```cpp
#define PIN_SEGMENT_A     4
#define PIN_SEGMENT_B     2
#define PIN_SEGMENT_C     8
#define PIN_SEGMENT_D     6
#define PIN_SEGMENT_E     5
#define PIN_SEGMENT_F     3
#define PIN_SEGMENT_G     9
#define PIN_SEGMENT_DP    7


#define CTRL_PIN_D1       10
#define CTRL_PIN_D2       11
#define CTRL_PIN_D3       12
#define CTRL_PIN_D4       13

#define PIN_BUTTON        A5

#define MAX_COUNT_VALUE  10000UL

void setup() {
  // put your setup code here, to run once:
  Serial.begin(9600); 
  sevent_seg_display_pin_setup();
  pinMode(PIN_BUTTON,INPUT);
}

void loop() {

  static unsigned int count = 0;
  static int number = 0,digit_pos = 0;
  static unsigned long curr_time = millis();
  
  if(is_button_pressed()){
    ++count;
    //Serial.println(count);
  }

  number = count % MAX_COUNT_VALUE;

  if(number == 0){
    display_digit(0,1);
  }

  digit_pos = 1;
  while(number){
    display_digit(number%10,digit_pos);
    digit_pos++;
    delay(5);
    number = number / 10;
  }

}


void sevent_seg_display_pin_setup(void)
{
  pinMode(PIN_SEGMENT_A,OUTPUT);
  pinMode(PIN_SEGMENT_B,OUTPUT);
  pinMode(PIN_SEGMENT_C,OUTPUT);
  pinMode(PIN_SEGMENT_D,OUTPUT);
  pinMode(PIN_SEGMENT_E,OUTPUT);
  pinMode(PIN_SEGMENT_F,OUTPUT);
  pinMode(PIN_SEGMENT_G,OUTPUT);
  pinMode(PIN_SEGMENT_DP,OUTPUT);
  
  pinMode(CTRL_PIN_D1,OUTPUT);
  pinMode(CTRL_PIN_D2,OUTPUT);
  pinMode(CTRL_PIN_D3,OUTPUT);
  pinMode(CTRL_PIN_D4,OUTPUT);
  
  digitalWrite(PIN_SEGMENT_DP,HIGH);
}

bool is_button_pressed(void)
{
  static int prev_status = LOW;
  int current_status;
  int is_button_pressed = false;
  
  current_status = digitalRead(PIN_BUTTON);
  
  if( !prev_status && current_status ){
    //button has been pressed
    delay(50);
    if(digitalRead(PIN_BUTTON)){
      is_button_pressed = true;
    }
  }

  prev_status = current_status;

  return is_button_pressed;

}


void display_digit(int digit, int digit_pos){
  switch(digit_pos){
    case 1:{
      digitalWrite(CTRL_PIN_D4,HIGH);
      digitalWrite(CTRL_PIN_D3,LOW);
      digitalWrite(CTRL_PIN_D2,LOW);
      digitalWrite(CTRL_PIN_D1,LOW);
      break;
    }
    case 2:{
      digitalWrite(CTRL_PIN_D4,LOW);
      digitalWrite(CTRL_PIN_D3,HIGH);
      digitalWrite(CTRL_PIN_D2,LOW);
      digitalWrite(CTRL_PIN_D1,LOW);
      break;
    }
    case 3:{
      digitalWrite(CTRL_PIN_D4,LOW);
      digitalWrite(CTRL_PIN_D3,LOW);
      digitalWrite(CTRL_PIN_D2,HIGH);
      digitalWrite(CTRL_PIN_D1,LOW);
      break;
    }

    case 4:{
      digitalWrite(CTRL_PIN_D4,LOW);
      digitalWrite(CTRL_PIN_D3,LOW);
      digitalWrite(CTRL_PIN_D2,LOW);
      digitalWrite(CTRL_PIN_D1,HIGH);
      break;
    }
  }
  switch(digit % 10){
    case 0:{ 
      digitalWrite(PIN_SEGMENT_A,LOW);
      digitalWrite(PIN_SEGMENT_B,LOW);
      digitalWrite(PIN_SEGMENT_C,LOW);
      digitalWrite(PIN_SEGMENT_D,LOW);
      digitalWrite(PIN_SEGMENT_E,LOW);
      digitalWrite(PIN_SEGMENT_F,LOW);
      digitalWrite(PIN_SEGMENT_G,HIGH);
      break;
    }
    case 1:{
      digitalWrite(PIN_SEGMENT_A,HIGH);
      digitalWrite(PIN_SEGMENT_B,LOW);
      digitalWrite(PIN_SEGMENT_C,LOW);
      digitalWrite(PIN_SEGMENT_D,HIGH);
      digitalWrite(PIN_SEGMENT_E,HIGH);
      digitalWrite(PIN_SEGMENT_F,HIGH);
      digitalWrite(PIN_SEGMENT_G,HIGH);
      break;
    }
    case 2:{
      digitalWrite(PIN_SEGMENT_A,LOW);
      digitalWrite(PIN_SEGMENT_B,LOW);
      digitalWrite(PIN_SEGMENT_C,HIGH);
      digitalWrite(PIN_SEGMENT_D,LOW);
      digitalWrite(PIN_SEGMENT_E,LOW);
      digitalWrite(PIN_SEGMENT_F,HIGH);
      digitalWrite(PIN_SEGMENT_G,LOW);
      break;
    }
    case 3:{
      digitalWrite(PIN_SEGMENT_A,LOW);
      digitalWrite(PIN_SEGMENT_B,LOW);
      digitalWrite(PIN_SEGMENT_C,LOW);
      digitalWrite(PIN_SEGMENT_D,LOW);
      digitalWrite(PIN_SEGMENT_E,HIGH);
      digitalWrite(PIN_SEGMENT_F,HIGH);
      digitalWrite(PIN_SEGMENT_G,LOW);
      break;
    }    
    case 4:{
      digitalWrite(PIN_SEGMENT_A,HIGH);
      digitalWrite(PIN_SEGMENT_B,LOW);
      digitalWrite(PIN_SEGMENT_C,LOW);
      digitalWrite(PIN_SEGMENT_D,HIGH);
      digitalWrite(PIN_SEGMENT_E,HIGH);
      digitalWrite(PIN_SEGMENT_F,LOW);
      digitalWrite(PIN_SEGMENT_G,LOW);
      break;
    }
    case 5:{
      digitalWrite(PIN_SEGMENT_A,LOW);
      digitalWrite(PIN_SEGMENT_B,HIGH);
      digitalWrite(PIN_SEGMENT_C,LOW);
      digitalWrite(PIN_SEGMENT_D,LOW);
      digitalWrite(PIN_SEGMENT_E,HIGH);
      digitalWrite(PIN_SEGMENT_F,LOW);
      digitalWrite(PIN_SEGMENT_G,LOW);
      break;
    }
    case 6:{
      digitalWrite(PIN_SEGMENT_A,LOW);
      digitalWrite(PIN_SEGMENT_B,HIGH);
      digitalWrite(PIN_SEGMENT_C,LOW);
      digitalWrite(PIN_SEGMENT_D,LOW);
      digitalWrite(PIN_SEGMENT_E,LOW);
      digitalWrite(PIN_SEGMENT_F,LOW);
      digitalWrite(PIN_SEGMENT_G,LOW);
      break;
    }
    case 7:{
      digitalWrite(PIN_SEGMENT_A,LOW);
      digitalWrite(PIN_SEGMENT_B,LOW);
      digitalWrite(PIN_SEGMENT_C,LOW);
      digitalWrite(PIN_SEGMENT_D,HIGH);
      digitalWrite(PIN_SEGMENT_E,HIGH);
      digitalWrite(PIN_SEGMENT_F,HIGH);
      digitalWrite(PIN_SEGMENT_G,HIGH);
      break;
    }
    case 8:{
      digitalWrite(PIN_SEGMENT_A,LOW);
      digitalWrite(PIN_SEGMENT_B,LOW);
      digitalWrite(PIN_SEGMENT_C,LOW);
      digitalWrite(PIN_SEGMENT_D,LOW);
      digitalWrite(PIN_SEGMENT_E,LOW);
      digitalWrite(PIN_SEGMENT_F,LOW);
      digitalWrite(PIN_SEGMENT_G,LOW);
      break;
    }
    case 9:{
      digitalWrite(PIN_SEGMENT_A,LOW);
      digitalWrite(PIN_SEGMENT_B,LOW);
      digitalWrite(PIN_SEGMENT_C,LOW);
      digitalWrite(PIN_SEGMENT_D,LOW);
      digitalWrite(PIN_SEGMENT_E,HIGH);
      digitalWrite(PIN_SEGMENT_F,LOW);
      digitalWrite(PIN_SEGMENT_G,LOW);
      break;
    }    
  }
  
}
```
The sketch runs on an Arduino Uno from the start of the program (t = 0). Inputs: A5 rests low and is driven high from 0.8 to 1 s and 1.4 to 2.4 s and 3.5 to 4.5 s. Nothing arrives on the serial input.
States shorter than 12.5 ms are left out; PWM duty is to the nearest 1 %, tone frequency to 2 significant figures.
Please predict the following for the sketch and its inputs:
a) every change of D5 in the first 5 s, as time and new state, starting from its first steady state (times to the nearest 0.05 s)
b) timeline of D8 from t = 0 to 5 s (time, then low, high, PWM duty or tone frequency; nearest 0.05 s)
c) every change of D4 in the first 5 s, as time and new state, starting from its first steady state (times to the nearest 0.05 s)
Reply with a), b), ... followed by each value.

a) 0 s low; 0.85 s high; 1.45 s low; 3.55 s high
b) 0 s low; 1.45 s high; 3.55 s low
c) 0 s low; 0.85 s high; 1.45 s low
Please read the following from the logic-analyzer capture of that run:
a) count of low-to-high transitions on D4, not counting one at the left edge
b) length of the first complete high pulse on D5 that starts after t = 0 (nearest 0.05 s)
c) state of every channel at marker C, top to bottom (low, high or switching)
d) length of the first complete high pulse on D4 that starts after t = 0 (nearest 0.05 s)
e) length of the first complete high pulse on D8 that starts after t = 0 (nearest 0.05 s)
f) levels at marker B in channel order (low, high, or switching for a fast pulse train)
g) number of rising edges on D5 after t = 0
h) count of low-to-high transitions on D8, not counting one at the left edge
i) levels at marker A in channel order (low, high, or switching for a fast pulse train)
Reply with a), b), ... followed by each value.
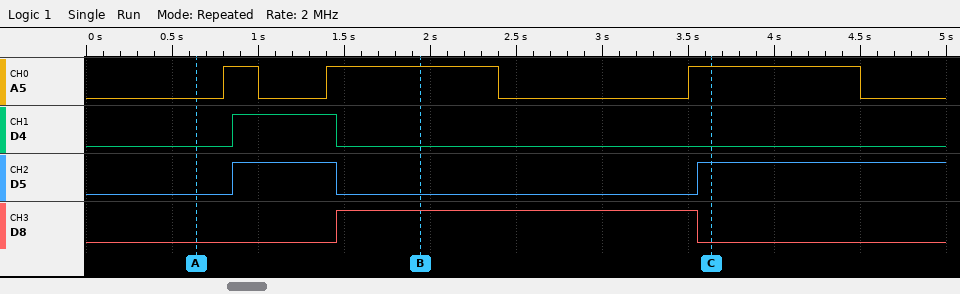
a) 1
b) 0.60 s
c) A5 high, D4 low, D5 high, D8 low
d) 0.60 s
e) 2.10 s
f) A5 high, D4 low, D5 low, D8 high
g) 2
h) 1
i) A5 low, D4 low, D5 low, D8 low
